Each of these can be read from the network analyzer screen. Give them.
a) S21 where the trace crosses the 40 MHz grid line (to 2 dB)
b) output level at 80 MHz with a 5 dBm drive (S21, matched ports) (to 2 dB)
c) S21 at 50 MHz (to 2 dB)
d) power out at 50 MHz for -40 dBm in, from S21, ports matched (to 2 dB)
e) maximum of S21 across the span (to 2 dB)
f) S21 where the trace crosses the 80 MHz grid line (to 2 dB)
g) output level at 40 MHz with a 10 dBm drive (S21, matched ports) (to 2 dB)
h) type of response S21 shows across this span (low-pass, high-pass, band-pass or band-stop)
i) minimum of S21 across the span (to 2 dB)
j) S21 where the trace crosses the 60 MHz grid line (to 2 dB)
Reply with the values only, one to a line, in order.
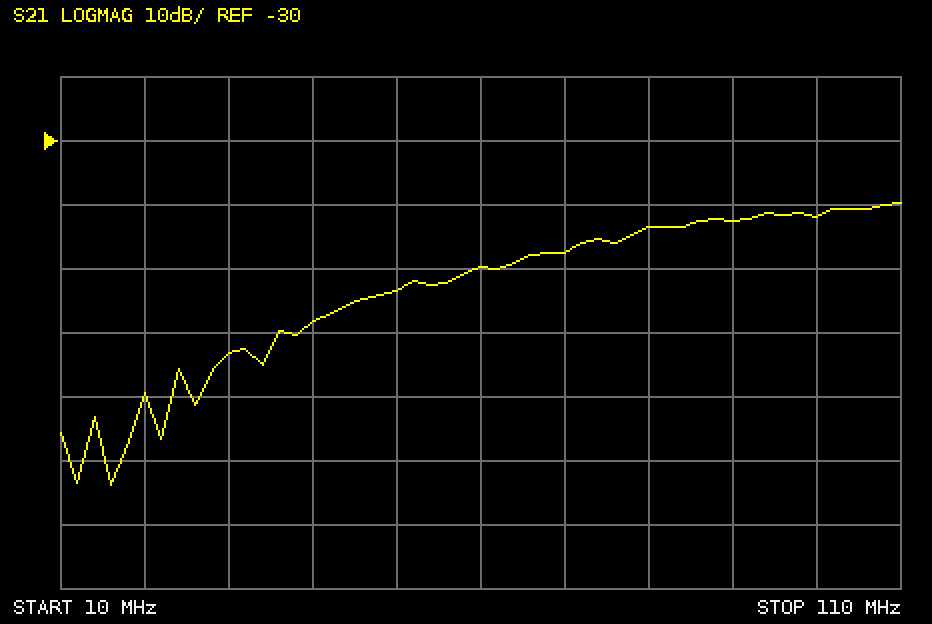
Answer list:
-58 dB
-38 dBm
-54 dB
-94 dBm
-40 dB
-44 dB
-48 dBm
high-pass
-84 dB
-50 dB
